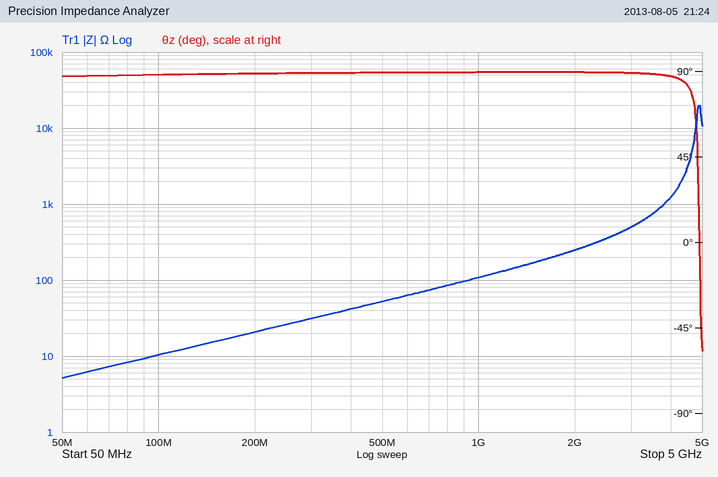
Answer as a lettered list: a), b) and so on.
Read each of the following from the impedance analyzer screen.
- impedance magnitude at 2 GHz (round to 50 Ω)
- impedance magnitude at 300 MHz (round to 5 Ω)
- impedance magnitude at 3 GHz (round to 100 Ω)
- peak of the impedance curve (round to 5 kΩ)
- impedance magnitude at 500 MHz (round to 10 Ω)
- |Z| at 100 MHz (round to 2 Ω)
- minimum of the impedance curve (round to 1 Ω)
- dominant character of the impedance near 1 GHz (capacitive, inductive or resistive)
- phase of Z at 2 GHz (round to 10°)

a) 250 Ω
b) 30 Ω
c) 500 Ω
d) 20 kΩ
e) 50 Ω
f) 10 Ω
g) 5 Ω
h) inductive
i) 90°
